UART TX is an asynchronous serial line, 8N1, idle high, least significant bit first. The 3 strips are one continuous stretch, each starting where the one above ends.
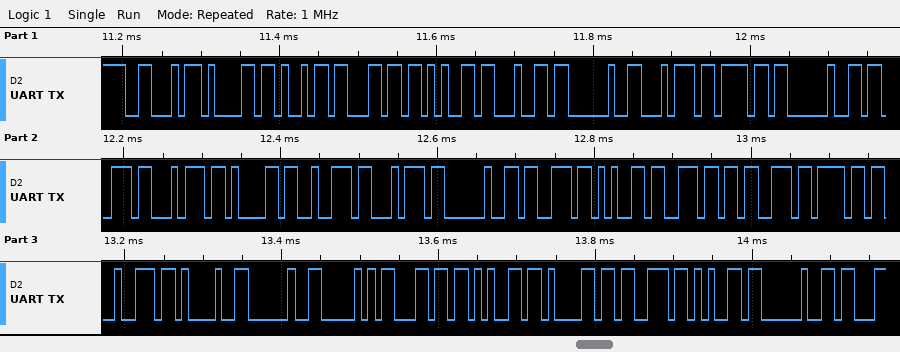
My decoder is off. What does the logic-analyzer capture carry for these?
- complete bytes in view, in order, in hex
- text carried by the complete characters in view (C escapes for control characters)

46 61 69 6C 65 64 20 74 6F 20 73 74 61 72 74 20 73 65 6E 73 6F 72 21 20 50 6C 65 61 73 65 20
"Failed to start sensor! Please "
